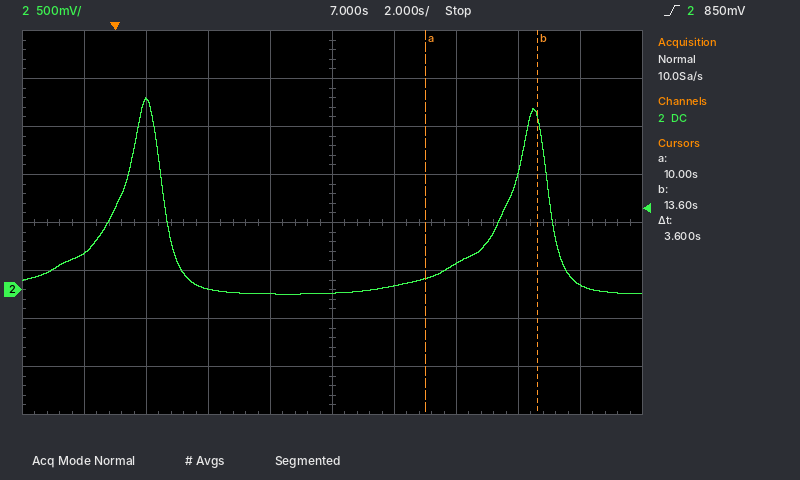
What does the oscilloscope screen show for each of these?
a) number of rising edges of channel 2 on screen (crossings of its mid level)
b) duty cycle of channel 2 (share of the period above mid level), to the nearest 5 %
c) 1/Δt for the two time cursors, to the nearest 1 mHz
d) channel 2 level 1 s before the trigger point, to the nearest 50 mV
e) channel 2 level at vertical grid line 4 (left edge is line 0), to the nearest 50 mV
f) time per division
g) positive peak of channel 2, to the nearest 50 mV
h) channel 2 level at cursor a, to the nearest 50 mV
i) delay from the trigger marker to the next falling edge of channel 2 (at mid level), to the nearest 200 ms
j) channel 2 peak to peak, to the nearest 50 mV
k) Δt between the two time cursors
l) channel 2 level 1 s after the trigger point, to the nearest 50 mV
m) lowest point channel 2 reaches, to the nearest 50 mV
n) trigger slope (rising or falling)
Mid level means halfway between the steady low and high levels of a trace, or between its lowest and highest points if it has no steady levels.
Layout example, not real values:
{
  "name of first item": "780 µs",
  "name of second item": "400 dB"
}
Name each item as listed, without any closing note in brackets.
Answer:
{
  "number of rising edges of channel 2 on screen": "2",
  "duty cycle of channel 2 (share of the period above mid level), to the nearest 5 %": "10 %",
  "1/Δt for the two time cursors, to the nearest 1 mHz": "278 mHz",
  "channel 2 level 1 s before the trigger point, to the nearest 50 mV": "400 mV",
  "channel 2 level at vertical grid line 4 (left edge is line 0), to the nearest 50 mV": "-50 mV",
  "time per division": "2 s",
  "positive peak of channel 2, to the nearest 50 mV": "2.00 V",
  "channel 2 level at cursor a, to the nearest 50 mV": "100 mV",
  "delay from the trigger marker to the next falling edge of channel 2 (at mid level), to the nearest 200 ms": "1.6 s",
  "channel 2 peak to peak, to the nearest 50 mV": "2.05 V",
  "Δt between the two time cursors": "3.6 s",
  "channel 2 level 1 s after the trigger point, to the nearest 50 mV": "1.95 V",
  "lowest point channel 2 reaches, to the nearest 50 mV": "-50 mV",
  "trigger slope": "rising"
}
